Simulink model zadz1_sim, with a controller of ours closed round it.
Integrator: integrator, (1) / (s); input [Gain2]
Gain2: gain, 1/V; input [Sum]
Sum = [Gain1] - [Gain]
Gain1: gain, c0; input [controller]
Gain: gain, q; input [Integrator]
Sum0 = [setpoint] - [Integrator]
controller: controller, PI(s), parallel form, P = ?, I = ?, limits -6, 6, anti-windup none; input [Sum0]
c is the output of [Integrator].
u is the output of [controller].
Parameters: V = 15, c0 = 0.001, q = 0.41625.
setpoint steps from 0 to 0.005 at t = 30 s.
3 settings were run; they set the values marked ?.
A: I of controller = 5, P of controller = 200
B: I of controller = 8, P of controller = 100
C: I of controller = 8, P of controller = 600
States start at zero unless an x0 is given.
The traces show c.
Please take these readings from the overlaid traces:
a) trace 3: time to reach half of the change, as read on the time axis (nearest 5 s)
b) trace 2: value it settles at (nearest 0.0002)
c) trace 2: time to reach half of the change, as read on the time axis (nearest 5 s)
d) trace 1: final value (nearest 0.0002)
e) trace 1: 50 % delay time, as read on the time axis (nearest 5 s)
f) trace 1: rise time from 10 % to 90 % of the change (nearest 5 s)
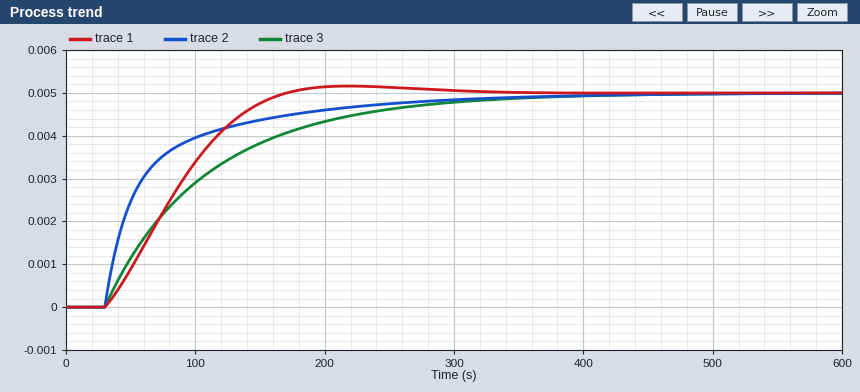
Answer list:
85 s
0.0050
50 s
0.0050
80 s
95 s
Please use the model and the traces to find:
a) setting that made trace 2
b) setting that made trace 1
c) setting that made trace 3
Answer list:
C
B
A
